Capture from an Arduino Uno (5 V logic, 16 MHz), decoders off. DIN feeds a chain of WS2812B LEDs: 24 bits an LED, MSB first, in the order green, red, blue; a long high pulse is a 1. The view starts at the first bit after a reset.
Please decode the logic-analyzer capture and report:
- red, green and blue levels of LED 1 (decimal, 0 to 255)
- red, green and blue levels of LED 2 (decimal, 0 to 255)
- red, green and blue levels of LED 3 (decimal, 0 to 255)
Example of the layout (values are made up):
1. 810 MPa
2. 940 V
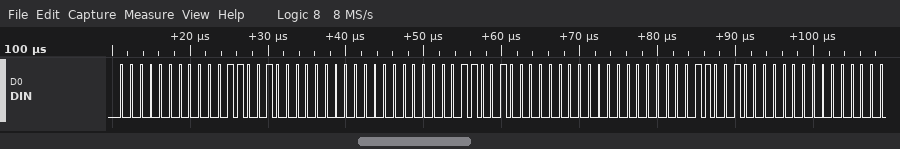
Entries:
1. 25, 0, 0
2. 25, 0, 0
3. 25, 0, 0
